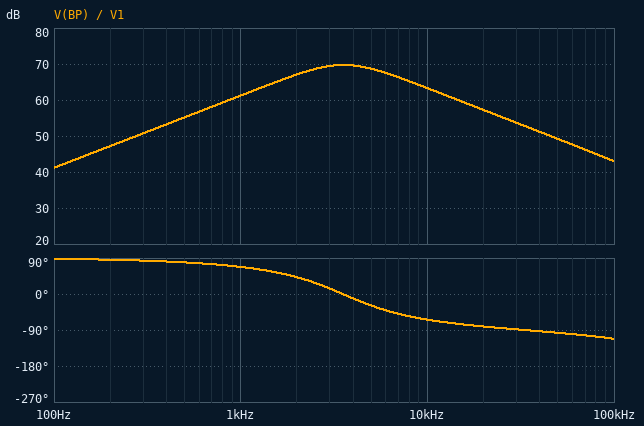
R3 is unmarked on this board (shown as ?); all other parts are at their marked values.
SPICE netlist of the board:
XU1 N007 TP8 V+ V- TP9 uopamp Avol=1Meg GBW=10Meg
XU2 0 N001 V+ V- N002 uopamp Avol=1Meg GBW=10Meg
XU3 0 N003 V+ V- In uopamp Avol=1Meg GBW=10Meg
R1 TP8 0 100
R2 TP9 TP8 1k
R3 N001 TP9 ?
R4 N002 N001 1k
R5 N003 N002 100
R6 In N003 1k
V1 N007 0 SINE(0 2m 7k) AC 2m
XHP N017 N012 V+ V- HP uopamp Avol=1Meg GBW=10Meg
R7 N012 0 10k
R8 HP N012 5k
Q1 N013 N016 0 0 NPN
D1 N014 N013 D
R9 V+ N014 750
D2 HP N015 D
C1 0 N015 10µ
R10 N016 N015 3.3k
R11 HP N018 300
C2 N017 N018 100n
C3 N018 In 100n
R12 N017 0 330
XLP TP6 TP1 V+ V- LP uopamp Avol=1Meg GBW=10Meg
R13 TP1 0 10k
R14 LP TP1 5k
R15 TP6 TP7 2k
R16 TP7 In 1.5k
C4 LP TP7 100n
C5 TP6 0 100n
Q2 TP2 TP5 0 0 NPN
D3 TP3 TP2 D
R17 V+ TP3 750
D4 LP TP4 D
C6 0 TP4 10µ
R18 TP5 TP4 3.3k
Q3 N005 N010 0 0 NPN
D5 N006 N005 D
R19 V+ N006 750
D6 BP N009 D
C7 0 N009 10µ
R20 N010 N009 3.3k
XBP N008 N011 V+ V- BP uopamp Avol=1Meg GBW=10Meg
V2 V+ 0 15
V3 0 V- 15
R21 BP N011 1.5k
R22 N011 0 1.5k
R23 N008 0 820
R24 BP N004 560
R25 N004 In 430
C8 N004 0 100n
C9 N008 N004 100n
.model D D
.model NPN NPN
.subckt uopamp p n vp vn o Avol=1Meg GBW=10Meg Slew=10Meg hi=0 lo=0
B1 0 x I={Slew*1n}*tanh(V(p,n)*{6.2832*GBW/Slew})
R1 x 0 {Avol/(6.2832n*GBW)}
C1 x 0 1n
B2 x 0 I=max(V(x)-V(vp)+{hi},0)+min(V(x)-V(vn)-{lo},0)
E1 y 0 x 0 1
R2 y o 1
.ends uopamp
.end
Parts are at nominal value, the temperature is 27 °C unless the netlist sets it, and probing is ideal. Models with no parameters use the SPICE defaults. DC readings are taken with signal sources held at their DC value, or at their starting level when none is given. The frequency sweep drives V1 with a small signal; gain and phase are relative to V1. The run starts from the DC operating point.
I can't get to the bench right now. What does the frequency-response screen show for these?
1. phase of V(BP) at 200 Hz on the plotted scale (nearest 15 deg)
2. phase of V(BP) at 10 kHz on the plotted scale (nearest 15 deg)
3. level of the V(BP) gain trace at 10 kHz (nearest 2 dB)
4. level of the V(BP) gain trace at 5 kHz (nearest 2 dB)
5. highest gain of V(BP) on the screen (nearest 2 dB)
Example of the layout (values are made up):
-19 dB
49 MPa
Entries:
90 deg
-60 deg
64 dB
68 dB
70 dB
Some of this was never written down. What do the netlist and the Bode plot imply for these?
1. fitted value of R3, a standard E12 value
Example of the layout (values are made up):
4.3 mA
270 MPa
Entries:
56 Ω
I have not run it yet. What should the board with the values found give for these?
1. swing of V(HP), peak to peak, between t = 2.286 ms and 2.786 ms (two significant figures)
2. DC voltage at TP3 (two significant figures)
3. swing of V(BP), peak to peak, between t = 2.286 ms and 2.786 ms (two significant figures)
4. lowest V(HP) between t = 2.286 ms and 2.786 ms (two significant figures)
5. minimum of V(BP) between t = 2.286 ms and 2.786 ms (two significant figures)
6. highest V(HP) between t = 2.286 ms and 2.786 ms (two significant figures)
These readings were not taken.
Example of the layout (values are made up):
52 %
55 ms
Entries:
11 V
15 V
8.3 V
-5.3 V
-4.1 V
5.3 V
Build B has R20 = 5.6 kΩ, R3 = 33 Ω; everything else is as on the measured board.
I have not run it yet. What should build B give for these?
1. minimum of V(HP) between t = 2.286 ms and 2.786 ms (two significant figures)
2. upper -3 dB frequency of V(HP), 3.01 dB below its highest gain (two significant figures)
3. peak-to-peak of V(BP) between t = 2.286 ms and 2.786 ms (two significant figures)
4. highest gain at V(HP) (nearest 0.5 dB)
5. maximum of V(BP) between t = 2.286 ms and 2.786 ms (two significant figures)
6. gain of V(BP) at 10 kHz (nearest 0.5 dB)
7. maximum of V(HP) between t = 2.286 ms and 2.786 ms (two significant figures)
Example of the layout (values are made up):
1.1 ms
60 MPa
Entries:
-9.0 V
260 kHz
14 V
74.0 dB
7.0 V
68.0 dB
9.0 V
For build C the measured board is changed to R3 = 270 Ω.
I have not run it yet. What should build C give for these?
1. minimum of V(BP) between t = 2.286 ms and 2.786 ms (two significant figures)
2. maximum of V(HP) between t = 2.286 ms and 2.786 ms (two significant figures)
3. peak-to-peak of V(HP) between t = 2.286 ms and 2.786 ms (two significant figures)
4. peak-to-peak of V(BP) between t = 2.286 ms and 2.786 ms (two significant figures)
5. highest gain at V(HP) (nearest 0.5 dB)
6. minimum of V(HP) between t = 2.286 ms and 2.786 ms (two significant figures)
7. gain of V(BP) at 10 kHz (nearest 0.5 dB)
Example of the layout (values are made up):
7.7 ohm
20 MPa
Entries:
-860 mV
1.1 V
2.2 V
1.7 V
55.5 dB
-1.1 V
49.5 dB
